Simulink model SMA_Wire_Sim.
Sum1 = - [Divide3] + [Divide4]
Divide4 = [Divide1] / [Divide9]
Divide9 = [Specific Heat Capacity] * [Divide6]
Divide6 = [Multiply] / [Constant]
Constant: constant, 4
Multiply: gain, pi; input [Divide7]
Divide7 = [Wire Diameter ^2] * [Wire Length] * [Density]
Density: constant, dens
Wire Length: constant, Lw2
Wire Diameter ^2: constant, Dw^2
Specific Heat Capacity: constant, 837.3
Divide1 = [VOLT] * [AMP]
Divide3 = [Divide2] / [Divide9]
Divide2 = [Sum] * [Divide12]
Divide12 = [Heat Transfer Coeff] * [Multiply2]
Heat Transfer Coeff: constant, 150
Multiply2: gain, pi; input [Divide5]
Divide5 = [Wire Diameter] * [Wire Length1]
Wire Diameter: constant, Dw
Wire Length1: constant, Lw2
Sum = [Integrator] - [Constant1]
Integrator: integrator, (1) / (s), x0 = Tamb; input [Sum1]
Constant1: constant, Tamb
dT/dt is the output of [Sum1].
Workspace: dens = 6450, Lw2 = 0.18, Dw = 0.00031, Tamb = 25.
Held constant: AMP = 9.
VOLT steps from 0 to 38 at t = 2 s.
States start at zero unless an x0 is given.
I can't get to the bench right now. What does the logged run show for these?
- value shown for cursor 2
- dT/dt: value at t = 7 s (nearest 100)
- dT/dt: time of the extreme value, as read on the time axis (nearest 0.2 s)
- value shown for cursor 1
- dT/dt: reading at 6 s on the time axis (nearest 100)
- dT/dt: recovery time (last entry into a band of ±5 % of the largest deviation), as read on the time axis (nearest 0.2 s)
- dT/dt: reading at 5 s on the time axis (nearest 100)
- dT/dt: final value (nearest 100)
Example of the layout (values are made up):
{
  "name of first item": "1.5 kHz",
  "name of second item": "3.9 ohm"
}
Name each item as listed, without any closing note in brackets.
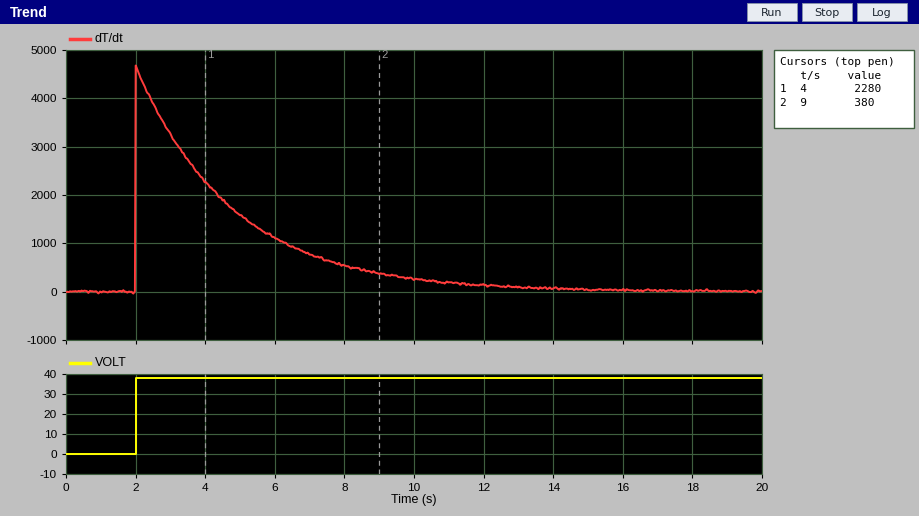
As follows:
{
  "value shown for cursor 2": "380",
  "dT/dt: value at t = 7 s": "800",
  "dT/dt: time of the extreme value, as read on the time axis": "2.0 s",
  "value shown for cursor 1": "2280",
  "dT/dt: reading at 6 s on the time axis": "1100",
  "dT/dt: recovery time (last entry into a band of ±5 % of the largest deviation), as read on the time axis": "10.4 s",
  "dT/dt: reading at 5 s on the time axis": "1600",
  "dT/dt: final value": "0"
}
